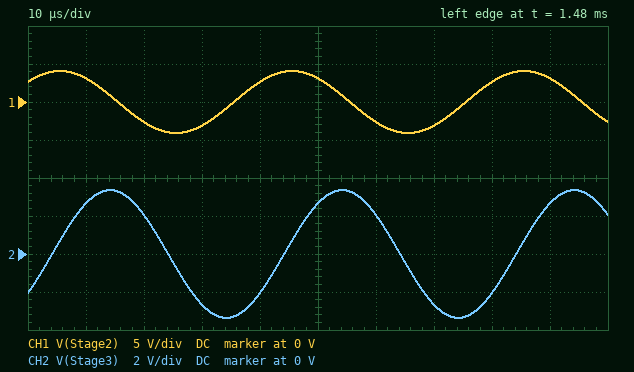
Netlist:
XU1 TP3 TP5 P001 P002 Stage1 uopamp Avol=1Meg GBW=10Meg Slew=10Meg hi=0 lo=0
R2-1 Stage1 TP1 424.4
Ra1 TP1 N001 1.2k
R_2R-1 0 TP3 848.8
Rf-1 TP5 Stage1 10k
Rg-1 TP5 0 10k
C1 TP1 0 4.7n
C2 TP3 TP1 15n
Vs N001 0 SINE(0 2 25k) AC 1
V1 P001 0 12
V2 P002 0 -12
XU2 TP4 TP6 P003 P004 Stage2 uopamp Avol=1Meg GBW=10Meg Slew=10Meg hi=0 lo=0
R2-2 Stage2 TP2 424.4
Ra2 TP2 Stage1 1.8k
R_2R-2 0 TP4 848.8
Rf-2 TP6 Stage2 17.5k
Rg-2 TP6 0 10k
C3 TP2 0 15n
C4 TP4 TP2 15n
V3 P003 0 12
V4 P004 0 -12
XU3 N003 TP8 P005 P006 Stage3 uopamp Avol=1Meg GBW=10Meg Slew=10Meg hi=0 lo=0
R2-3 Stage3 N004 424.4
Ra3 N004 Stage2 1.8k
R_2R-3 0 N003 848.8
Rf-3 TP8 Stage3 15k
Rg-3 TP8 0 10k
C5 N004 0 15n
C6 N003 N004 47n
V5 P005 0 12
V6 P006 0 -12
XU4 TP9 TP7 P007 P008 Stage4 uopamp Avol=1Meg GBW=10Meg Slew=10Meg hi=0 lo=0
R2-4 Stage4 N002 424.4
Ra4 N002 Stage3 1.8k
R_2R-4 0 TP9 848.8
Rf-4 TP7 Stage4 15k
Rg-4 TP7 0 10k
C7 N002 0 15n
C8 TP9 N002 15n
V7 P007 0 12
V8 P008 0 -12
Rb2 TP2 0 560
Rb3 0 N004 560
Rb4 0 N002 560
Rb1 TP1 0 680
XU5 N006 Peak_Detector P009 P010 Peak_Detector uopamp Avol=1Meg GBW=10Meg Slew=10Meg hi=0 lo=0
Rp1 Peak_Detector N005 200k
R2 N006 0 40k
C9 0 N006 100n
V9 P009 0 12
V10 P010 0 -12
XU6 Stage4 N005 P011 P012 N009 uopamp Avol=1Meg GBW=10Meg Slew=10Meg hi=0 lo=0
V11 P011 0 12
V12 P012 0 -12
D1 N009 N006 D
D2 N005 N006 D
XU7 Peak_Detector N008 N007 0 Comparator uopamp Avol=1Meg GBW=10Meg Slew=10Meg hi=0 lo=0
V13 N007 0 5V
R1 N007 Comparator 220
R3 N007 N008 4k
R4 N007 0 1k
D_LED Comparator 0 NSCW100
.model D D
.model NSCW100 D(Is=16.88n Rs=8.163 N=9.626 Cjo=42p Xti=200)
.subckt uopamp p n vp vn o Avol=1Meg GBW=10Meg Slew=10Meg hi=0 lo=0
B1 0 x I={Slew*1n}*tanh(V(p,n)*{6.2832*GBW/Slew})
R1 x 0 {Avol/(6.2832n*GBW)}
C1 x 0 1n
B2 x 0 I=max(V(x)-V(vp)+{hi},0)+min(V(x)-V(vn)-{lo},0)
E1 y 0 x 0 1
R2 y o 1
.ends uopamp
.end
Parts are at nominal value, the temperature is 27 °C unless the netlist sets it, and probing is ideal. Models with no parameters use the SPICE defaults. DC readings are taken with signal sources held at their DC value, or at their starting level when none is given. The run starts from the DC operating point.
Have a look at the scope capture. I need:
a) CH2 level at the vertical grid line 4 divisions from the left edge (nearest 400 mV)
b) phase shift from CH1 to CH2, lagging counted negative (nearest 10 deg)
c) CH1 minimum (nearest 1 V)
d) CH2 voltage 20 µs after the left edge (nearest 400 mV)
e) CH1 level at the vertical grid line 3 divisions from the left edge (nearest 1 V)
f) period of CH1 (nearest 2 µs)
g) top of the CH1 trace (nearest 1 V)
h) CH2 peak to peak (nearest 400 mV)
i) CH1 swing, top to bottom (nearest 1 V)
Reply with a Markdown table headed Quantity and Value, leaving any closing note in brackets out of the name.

| Quantity | Value |
|---|---|
| CH2 level at the vertical grid line 4 divisions from the left edge | -2.0 V |
| phase shift from CH1 to CH2, lagging counted negative | -80 deg |
| CH1 minimum | -4 V |
| CH2 voltage 20 µs after the left edge | 2.0 V |
| CH1 level at the vertical grid line 3 divisions from the left edge | -3 V |
| period of CH1 | 40 µs |
| top of the CH1 trace | 4 V |
| CH2 peak to peak | 6.8 V |
| CH1 swing, top to bottom | 8 V |
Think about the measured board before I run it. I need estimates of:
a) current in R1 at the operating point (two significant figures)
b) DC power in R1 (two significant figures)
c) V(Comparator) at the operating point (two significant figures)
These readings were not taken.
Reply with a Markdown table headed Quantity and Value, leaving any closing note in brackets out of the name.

| Quantity | Value |
|---|---|
| current in R1 at the operating point | 23 mA |
| DC power in R1 | 110 mW |
| V(Comparator) at the operating point | 13 mV |
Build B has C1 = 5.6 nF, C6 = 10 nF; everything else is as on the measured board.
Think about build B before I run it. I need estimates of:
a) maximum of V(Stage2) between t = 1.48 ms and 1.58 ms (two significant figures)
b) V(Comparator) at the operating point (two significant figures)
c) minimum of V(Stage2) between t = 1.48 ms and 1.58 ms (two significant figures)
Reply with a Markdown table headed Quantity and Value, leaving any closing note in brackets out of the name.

| Quantity | Value |
|---|---|
| maximum of V(Stage2) between t = 1.48 ms and 1.58 ms | 4.2 V |
| V(Comparator) at the operating point | 13 mV |
| minimum of V(Stage2) between t = 1.48 ms and 1.58 ms | -4.2 V |
